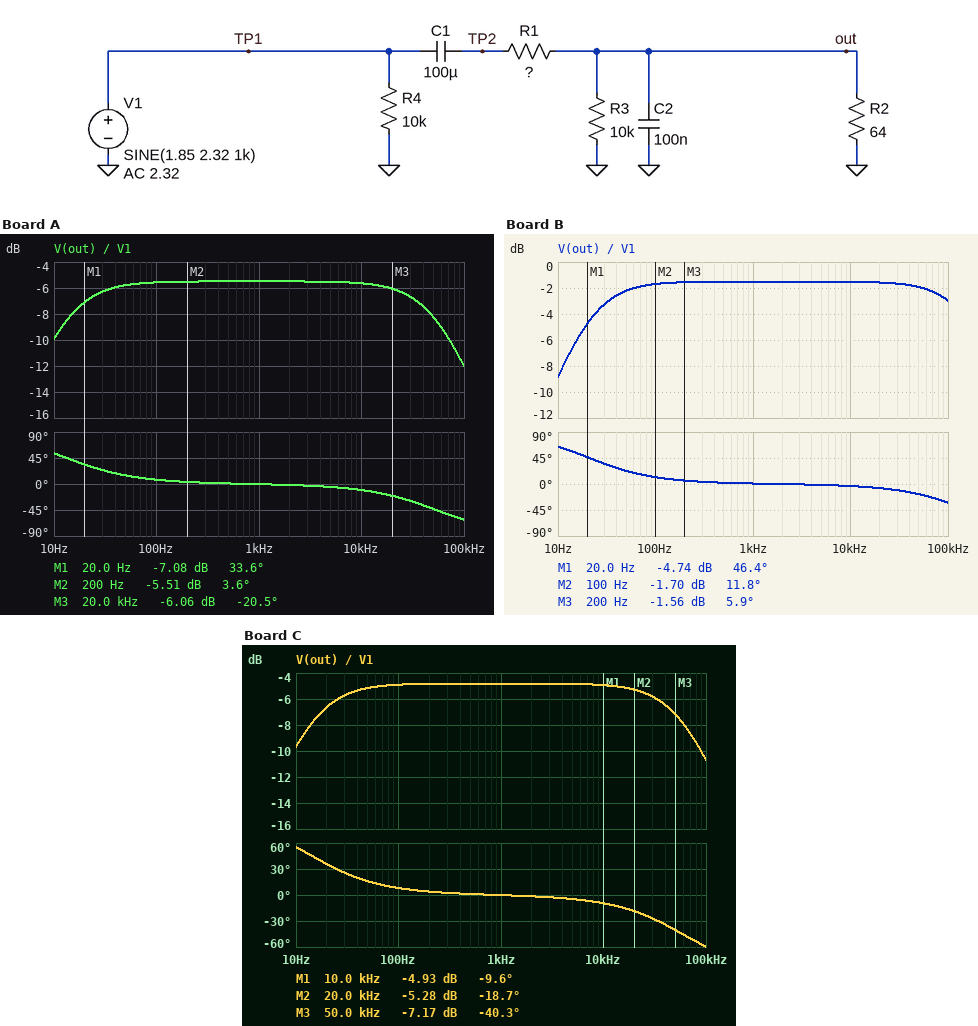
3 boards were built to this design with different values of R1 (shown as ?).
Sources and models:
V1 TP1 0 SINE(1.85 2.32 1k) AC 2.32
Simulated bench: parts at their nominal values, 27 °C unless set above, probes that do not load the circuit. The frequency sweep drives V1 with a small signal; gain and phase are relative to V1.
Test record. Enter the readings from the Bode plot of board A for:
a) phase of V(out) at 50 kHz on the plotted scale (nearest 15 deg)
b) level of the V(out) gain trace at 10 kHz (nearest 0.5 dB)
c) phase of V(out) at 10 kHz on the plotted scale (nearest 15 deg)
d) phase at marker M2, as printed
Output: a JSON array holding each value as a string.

["-45 deg", "-5.5 dB", "-15 deg", "3.6 deg"]
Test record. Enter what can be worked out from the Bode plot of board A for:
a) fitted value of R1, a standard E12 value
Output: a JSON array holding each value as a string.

["56 Ω"]
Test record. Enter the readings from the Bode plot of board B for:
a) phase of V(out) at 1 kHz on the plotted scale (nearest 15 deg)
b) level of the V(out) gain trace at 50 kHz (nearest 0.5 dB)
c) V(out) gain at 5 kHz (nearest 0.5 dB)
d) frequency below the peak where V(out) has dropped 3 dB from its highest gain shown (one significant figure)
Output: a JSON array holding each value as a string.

["0 deg", "-2.0 dB", "-1.5 dB", "20 Hz"]
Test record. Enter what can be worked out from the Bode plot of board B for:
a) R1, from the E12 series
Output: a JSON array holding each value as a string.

["12 Ω"]
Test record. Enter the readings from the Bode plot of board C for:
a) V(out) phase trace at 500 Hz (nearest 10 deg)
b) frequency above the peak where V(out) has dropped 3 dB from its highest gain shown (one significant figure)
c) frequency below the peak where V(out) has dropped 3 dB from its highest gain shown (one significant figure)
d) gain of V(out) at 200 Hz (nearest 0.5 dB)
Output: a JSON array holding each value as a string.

["0 deg", "60 kHz", "10 Hz", "-5.0 dB"]
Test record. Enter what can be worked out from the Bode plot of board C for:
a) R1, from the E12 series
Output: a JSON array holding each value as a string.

["47 Ω"]
